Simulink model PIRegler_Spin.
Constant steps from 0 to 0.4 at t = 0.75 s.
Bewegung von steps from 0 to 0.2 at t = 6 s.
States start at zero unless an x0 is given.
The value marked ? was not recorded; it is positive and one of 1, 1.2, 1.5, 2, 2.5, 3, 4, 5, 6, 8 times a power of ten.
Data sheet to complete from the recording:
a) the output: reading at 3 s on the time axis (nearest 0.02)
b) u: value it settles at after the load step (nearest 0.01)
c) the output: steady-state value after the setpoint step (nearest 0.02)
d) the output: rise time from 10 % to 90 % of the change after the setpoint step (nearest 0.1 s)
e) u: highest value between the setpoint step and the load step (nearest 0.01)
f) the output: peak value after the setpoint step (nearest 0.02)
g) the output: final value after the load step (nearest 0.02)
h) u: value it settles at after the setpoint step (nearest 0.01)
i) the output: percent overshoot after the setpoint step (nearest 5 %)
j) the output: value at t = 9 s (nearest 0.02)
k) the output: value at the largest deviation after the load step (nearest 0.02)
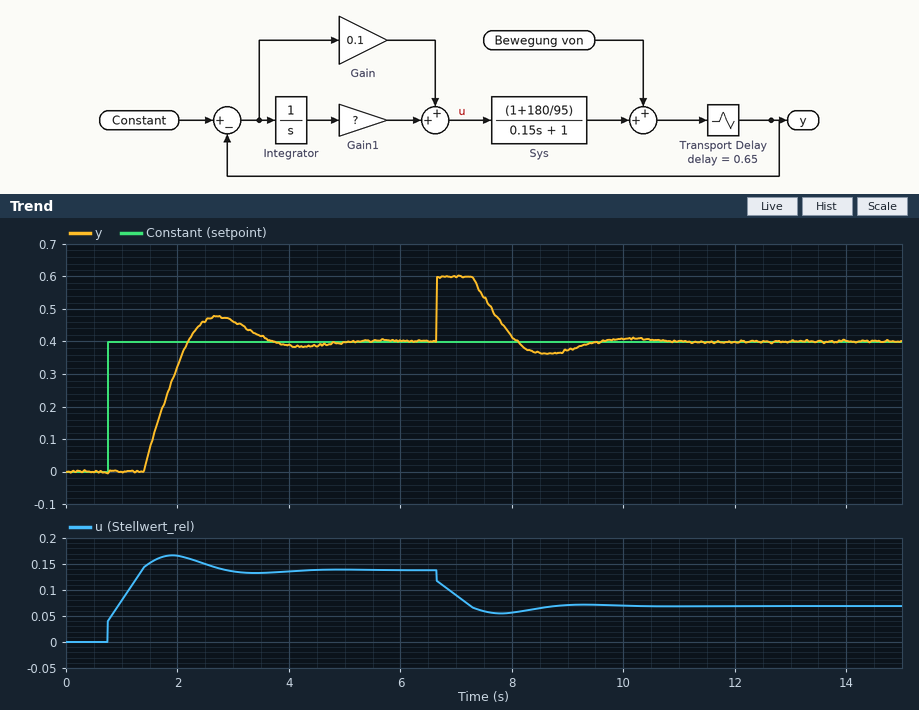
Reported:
0.46
0.07
0.40
0.6 s
0.17
0.48
0.40
0.14
20 %
0.38
0.60
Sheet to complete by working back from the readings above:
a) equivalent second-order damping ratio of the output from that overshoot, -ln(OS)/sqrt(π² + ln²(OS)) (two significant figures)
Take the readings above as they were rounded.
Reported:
0.46
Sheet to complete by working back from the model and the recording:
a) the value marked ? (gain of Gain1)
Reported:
0.4
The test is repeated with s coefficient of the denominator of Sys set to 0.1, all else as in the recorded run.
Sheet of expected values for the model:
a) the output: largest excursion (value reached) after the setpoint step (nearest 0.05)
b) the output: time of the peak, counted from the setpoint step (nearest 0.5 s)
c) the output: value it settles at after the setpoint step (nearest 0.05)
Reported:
0.45
2.0 s
0.40
